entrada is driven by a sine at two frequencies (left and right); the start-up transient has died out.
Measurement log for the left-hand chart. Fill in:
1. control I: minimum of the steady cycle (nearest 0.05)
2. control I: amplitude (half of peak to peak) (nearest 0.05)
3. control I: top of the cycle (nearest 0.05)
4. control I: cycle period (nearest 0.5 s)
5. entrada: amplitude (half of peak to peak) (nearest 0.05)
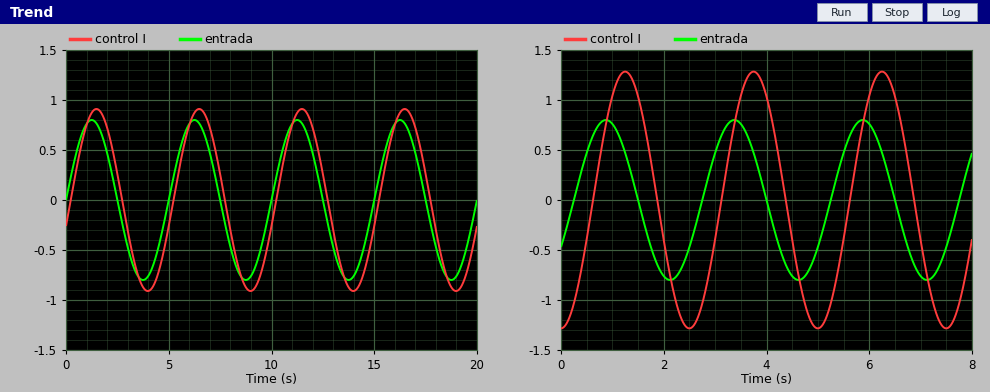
-0.90
0.90
0.90
5.0 s
0.80
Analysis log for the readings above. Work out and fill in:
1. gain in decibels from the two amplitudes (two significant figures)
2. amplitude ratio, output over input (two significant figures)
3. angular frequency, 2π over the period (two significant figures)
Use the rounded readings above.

1.0 dB
1.1
1.3 rad/s
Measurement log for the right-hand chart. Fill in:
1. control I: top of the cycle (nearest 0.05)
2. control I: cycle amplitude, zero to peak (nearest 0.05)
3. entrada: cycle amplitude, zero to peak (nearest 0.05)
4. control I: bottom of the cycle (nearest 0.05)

1.30
1.30
0.80
-1.30
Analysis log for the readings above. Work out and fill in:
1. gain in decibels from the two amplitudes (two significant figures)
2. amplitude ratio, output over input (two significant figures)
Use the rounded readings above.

4.2 dB
1.6
